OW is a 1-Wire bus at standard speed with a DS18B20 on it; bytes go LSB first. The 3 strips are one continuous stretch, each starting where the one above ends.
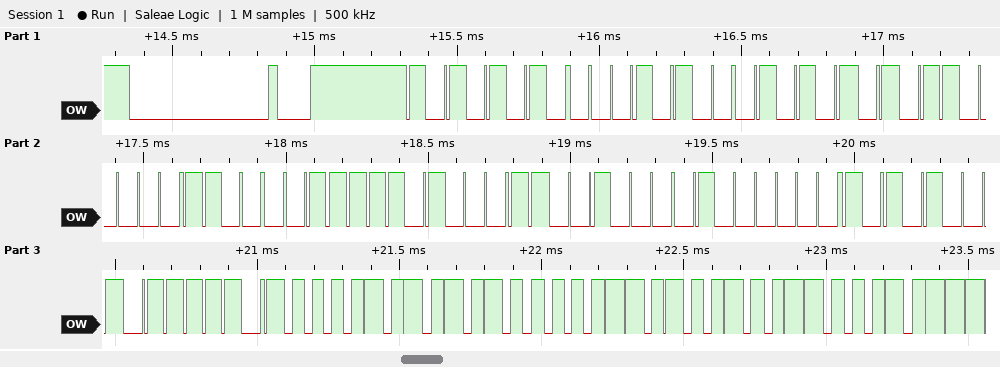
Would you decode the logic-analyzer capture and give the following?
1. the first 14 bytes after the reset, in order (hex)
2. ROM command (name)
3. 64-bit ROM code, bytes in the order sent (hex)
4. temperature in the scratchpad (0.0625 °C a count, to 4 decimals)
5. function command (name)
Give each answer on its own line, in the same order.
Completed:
55 28 AA 06 C3 17 13 02 95 BE 50 05 4B 46
Match ROM
28 AA 06 C3 17 13 02 95
85.0000 °C
Read Scratchpad
